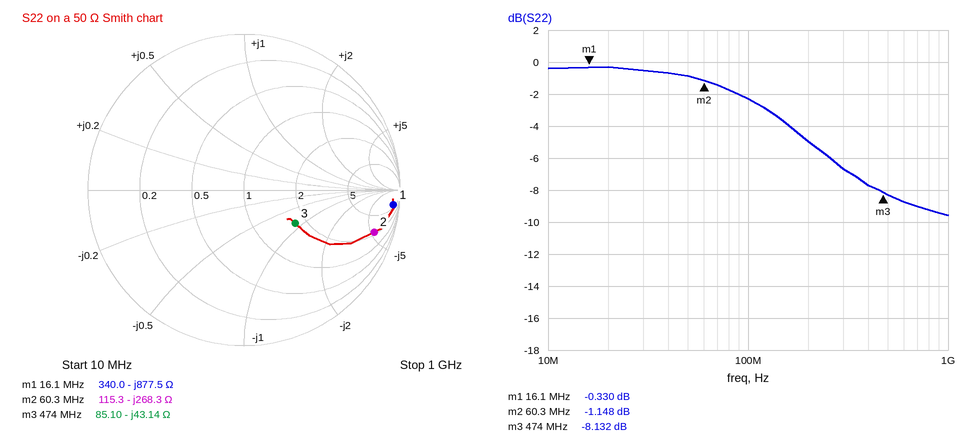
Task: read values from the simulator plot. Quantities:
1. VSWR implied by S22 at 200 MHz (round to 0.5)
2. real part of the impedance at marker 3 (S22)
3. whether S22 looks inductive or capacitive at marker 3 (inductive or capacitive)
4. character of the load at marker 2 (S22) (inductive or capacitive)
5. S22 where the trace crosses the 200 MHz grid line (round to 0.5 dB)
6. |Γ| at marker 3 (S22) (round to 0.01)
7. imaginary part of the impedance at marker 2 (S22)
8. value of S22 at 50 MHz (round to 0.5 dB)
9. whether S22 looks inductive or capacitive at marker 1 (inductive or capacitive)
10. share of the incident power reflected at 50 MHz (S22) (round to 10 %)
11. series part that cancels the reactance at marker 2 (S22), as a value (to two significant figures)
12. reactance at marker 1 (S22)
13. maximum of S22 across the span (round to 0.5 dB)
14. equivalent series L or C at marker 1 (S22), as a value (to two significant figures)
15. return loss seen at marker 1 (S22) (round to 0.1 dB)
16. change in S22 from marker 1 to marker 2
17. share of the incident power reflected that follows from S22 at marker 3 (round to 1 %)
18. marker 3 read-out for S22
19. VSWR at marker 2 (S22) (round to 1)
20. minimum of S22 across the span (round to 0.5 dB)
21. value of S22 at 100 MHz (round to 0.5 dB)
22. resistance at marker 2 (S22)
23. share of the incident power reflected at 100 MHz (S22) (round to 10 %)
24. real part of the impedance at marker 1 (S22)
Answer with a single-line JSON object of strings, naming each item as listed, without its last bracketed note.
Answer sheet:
{"VSWR implied by S22 at 200 MHz": "3.5", "real part of the impedance at marker 3": "85.10 Ω", "whether S22 looks inductive or capacitive at marker 3": "capacitive", "character of the load at marker 2 (S22)": "capacitive", "S22 where the trace crosses the 200 MHz grid line": "-5.0 dB", "|Γ| at marker 3 (S22)": "0.39", "imaginary part of the impedance at marker 2": "-268.3 Ω", "value of S22 at 50 MHz": "-1.0 dB", "whether S22 looks inductive or capacitive at marker 1": "capacitive", "share of the incident power reflected at 50 MHz (S22)": "80 %", "series part that cancels the reactance at marker 2 (S22), as a value": "710 nH", "reactance at marker 1": "-877.5 Ω", "maximum of S22 across the span": "-0.5 dB", "equivalent series L or C at marker 1 (S22), as a value": "11 pF", "return loss seen at marker 1 (S22)": "0.3 dB", "change in S22 from marker 1 to marker 2": "-0.818 dB", "share of the incident power reflected that follows from S22 at marker 3": "15 %", "marker 3 read-out for S22": "-8.132 dB", "VSWR at marker 2 (S22)": "15", "minimum of S22 across the span": "-9.5 dB", "value of S22 at 100 MHz": "-2.5 dB", "resistance at marker 2": "115.3 Ω", "share of the incident power reflected at 100 MHz (S22)": "60 %", "real part of the impedance at marker 1": "340.0 Ω"}
